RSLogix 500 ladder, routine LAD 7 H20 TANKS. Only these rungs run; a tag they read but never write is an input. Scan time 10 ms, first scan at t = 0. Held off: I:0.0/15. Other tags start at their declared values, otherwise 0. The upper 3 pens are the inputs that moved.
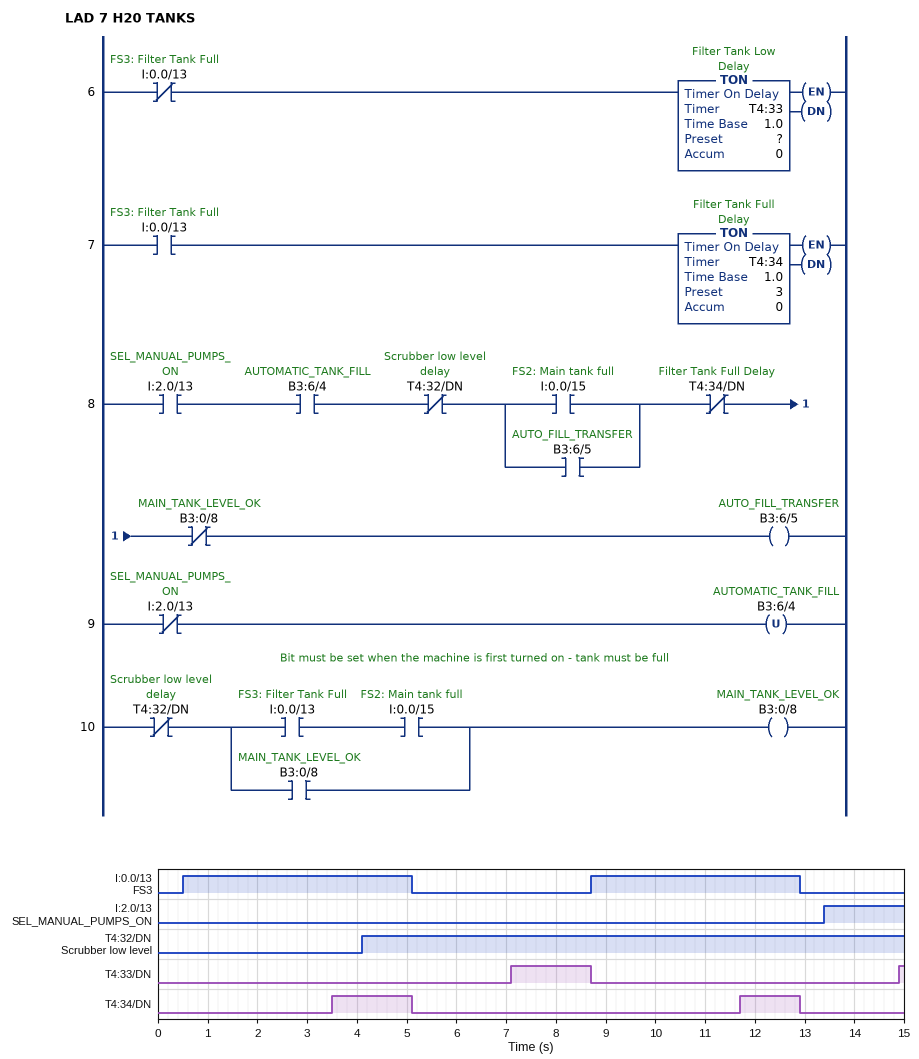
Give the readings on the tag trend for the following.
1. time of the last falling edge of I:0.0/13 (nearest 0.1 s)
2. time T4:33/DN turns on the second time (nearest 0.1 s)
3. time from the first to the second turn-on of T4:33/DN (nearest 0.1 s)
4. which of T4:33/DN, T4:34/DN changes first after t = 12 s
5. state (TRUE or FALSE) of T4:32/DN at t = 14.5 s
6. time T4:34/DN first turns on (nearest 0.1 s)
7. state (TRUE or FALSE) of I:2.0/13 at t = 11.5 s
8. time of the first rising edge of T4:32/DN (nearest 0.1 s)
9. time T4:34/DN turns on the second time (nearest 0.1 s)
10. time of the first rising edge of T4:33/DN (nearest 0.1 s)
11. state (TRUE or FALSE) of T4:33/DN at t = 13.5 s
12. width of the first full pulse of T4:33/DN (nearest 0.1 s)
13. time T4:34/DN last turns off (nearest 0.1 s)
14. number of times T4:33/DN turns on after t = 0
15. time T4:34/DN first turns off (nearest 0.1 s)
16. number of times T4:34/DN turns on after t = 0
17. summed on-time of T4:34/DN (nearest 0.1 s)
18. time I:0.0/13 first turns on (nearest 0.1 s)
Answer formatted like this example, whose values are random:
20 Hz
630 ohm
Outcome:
12.9 s
14.9 s
7.8 s
T4:34/DN
TRUE
3.5 s
FALSE
4.1 s
11.7 s
7.1 s
FALSE
1.6 s
12.9 s
2
5.1 s
2
2.8 s
0.5 s
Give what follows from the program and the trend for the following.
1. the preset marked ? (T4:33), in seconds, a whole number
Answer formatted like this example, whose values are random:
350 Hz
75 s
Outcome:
2 s
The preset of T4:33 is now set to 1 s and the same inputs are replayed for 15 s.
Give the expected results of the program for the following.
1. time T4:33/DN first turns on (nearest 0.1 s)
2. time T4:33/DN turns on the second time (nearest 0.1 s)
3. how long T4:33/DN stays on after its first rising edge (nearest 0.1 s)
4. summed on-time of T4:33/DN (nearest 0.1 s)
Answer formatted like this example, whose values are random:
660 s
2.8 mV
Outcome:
6.1 s
13.9 s
2.6 s
3.7 s
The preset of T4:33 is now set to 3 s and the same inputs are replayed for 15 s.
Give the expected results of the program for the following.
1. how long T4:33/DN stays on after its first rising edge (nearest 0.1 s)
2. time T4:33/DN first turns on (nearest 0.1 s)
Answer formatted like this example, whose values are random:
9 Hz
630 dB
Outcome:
0.6 s
8.1 s
